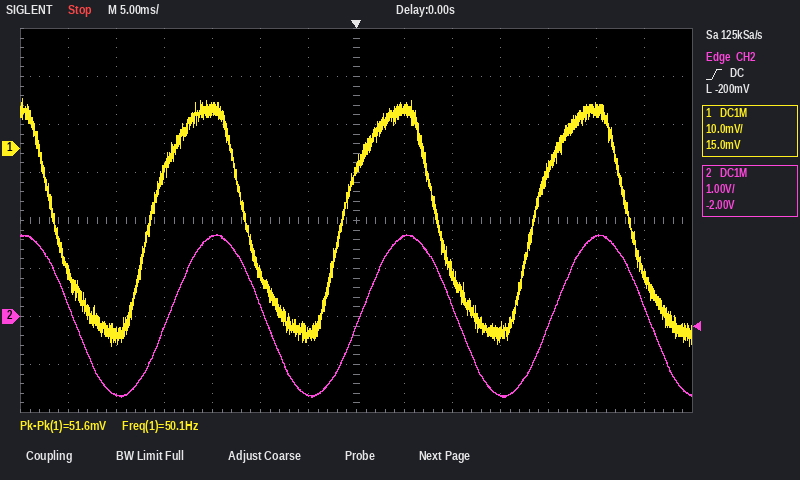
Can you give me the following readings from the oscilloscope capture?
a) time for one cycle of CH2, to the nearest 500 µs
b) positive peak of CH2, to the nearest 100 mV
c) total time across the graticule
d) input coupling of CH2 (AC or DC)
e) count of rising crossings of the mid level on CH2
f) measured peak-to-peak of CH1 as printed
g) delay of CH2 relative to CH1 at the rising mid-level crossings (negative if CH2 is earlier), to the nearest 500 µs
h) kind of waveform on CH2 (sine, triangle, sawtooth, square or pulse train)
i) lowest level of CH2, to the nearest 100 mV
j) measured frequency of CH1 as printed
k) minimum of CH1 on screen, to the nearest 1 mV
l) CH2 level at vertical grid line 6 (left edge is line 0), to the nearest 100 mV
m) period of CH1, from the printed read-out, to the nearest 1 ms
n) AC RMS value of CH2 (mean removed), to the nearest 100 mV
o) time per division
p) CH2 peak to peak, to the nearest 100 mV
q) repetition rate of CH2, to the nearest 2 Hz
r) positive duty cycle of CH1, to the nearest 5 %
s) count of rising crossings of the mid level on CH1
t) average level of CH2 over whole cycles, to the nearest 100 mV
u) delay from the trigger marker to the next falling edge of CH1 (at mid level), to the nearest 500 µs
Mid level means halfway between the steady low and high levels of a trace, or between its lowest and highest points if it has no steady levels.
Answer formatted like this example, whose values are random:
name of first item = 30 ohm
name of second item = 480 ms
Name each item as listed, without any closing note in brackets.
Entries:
time for one cycle of CH2, to the nearest 500 µs = 20.0 ms
positive peak of CH2, to the nearest 100 mV = 1.7 V
total time across the graticule = 70 ms
input coupling of CH2 = DC
count of rising crossings of the mid level on CH2 = 3
measured peak-to-peak of CH1 as printed = 51.6 mV
delay of CH2 relative to CH1 at the rising mid-level crossings (negative if CH2 is earlier), to the nearest 500 µs = +2.0 ms
kind of waveform on CH2 = sine
lowest level of CH2, to the nearest 100 mV = -1.7 V
measured frequency of CH1 as printed = 50.1 Hz
minimum of CH1 on screen, to the nearest 1 mV = -41 mV
CH2 level at vertical grid line 6 (left edge is line 0), to the nearest 100 mV = -1.6 V
period of CH1, from the printed read-out, to the nearest 1 ms = 20 ms
AC RMS value of CH2 (mean removed), to the nearest 100 mV = 1.2 V
time per division = 5 ms
CH2 peak to peak, to the nearest 100 mV = 3.4 V
repetition rate of CH2, to the nearest 2 Hz = 50 Hz
positive duty cycle of CH1, to the nearest 5 % = 50 %
count of rising crossings of the mid level on CH1 = 3
average level of CH2 over whole cycles, to the nearest 100 mV = 0.0 V
delay from the trigger marker to the next falling edge of CH1 (at mid level), to the nearest 500 µs = 8.5 ms
